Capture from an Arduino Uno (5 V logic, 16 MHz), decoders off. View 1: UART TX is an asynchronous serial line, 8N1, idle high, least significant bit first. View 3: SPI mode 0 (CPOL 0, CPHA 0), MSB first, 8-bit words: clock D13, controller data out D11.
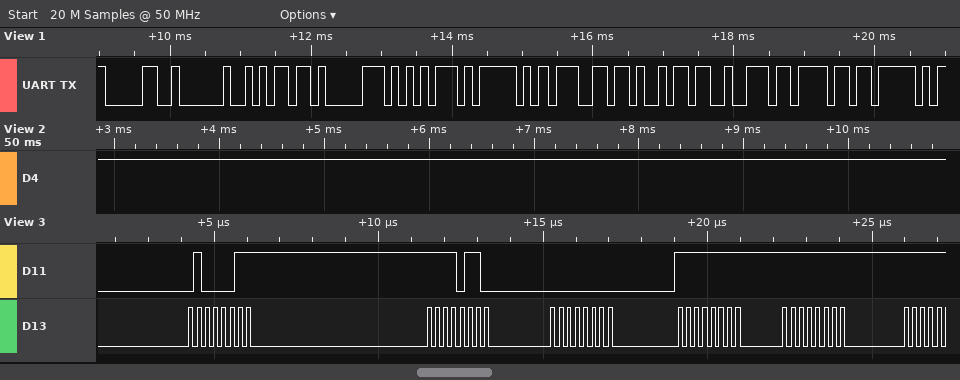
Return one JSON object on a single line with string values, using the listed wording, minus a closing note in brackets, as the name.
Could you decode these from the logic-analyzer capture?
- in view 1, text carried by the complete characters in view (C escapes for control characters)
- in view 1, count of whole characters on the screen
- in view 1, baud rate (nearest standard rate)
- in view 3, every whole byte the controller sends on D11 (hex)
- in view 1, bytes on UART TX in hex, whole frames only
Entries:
{"in view 1, text carried by the complete characters in view": "\"0 mpu_giro_\"", "in view 1, count of whole characters on the screen": "11", "in view 1, baud rate": "9600 baud", "in view 3, every whole byte the controller sends on D11": "43 F6 00 FF FF", "in view 1, bytes on UART TX in hex, whole frames only": "30 20 6D 70 75 5F 67 69 72 6F 5F"}
